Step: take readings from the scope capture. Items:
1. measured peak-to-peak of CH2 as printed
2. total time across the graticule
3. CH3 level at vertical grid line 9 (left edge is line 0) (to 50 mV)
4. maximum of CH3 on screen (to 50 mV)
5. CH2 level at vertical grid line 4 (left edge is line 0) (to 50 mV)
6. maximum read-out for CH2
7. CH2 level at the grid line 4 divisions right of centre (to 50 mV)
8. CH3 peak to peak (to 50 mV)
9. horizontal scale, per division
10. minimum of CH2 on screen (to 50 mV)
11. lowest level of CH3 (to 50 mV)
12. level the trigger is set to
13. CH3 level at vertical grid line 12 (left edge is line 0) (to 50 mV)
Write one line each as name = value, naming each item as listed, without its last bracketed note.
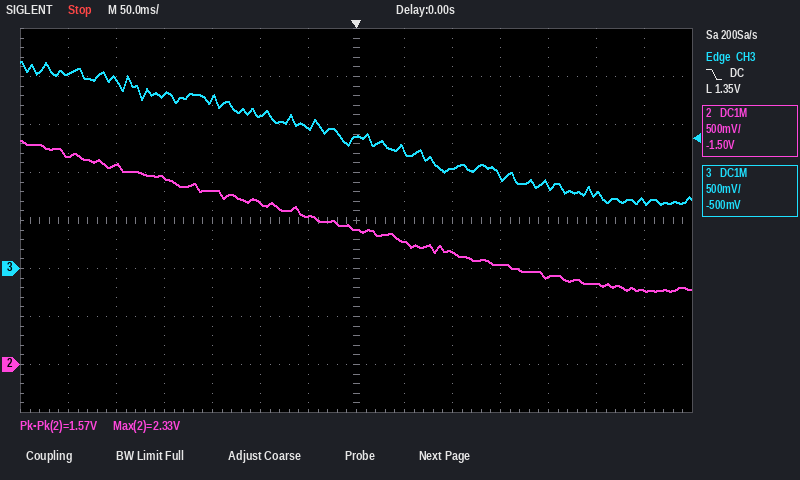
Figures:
measured peak-to-peak of CH2 as printed = 1.57 V
total time across the graticule = 700 ms
CH3 level at vertical grid line 9 (left edge is line 0) = 1.05 V
maximum of CH3 on screen = 2.15 V
CH2 level at vertical grid line 4 (left edge is line 0) = 1.80 V
maximum read-out for CH2 = 2.33 V
CH2 level at the grid line 4 divisions right of centre = 900 mV
CH3 peak to peak = 1.50 V
horizontal scale, per division = 50 ms
minimum of CH2 on screen = 750 mV
lowest level of CH3 = 650 mV
level the trigger is set to = 1.35 V
CH3 level at vertical grid line 12 (left edge is line 0) = 800 mV
